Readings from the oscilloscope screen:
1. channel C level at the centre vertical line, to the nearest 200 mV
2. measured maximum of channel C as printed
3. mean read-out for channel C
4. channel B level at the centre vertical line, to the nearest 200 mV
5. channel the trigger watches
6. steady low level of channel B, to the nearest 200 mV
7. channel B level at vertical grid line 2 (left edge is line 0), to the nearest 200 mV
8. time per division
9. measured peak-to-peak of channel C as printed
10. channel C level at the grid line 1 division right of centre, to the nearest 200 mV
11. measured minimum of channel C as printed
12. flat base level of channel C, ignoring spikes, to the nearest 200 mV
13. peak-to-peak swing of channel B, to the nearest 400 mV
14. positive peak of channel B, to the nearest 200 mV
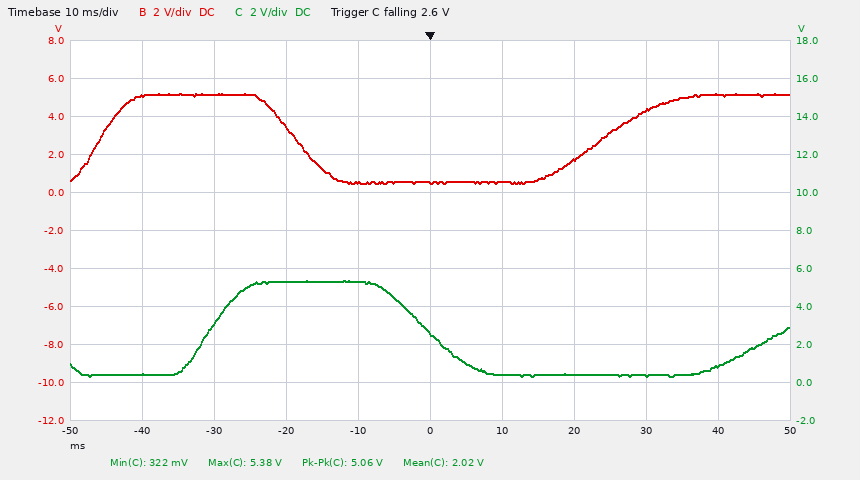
2.6 V
5.38 V
2.02 V
600 mV
channel C
600 mV
5.2 V
10 ms
5.06 V
400 mV
322 mV
400 mV
4.8 V
5.2 V
